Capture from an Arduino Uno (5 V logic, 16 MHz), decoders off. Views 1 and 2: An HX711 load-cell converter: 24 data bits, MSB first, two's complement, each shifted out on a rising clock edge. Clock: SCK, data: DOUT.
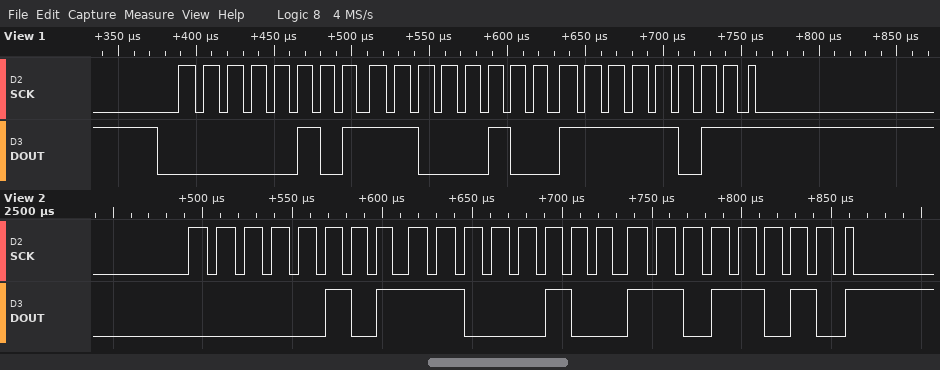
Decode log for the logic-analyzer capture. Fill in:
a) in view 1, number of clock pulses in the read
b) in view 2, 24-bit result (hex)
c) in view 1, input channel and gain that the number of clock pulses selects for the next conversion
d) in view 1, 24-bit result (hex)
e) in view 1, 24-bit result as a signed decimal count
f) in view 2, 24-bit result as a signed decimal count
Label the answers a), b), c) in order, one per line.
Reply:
a) 25
b) 0x05C4DA
c) channel A, gain 128
d) 0x05C4FB
e) 378107
f) 378074
